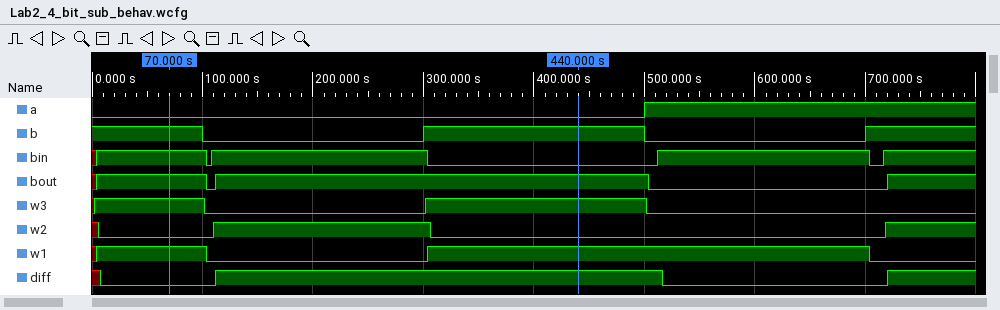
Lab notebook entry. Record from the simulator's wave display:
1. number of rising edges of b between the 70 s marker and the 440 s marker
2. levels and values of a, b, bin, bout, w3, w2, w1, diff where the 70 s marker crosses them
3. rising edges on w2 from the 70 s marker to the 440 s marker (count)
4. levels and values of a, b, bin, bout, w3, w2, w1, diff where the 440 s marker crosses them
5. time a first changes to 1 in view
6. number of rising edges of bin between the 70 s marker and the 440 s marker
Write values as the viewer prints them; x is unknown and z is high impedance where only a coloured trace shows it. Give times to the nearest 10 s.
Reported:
1
a=0, b=1, bin=1, bout=1, w3=1, w2=0, w1=1, diff=0
1
a=0, b=1, bin=0, bout=1, w3=1, w2=0, w1=1, diff=1
500 s
1
